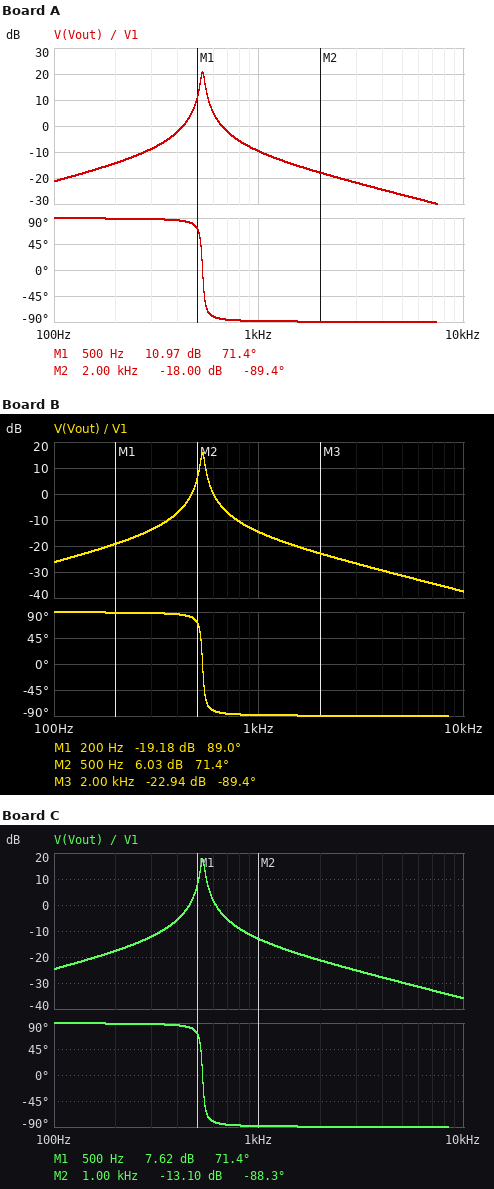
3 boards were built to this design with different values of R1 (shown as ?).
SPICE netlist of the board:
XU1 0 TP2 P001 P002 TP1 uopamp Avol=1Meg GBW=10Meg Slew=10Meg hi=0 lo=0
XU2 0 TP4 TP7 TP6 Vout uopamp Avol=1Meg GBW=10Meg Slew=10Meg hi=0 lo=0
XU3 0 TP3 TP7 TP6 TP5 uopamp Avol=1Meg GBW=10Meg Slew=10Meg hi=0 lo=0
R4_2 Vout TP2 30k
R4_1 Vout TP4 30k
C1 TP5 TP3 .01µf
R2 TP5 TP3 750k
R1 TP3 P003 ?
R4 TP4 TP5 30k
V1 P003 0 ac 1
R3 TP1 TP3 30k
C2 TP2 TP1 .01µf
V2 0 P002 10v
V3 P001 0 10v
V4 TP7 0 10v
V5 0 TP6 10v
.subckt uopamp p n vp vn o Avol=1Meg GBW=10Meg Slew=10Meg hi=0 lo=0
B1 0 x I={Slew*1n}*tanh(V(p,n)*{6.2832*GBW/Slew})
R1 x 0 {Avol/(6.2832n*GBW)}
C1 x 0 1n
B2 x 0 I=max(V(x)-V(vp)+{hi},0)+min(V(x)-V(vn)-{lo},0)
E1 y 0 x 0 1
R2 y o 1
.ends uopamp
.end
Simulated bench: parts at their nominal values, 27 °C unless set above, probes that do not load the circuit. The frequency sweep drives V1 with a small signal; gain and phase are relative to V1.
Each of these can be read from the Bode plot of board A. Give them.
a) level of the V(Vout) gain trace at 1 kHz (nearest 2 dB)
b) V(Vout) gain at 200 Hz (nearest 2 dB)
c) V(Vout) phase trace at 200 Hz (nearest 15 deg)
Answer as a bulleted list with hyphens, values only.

- -10 dB
- -14 dB
- 90 deg
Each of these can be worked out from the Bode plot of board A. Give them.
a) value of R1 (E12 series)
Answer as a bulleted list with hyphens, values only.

- 68 kΩ
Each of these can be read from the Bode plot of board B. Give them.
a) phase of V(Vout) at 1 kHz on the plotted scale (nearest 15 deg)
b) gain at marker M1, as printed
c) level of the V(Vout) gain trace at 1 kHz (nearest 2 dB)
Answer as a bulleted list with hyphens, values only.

- -90 deg
- -19.18 dB
- -14 dB
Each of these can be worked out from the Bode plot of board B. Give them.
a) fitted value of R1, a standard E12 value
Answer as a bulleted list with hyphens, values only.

- 120 kΩ
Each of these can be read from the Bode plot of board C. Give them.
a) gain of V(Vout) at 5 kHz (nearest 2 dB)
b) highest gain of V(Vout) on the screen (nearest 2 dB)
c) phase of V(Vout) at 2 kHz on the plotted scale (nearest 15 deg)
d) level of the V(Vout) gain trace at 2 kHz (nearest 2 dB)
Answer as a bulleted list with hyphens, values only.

- -30 dB
- 18 dB
- -90 deg
- -22 dB
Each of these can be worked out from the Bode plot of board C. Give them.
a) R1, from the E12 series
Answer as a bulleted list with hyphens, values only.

- 100 kΩ
